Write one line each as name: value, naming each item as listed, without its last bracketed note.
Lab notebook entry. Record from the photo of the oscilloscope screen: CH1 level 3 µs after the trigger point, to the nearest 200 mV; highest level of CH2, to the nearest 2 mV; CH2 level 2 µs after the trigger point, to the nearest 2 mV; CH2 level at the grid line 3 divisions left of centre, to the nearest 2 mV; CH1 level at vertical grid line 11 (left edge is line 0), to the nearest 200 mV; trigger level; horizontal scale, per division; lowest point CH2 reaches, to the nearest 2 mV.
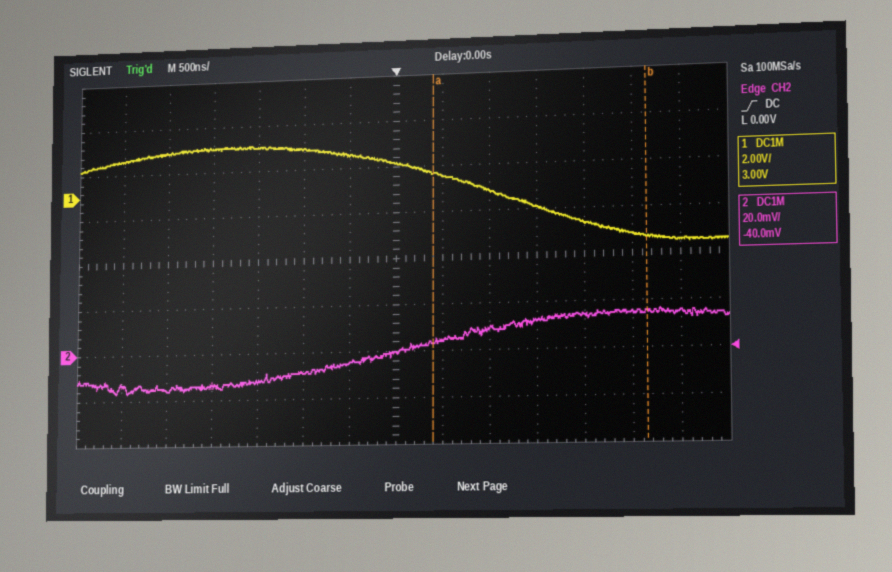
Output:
CH1 level 3 µs after the trigger point, to the nearest 200 mV: -2.4 V
highest level of CH2, to the nearest 2 mV: 16 mV
CH2 level 2 µs after the trigger point, to the nearest 2 mV: 14 mV
CH2 level at the grid line 3 divisions left of centre, to the nearest 2 mV: -12 mV
CH1 level at vertical grid line 11 (left edge is line 0), to the nearest 200 mV: -1.6 V
trigger level: 0.00 V
horizontal scale, per division: 500 ns
lowest point CH2 reaches, to the nearest 2 mV: -16 mV
